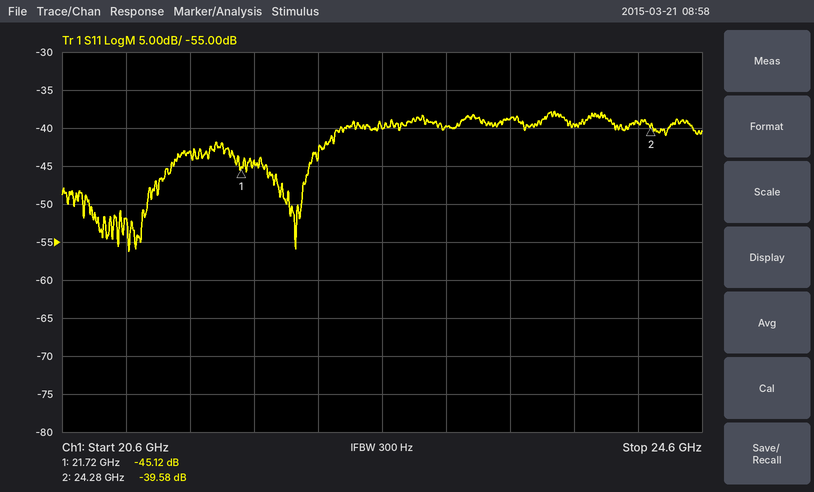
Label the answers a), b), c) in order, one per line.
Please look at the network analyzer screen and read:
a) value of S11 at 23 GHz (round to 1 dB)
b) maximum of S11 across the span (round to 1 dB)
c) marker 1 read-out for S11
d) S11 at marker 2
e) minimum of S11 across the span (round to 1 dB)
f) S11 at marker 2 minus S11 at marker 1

a) -40 dB
b) -38 dB
c) -45.12 dB
d) -39.58 dB
e) -56 dB
f) 5.54 dB
